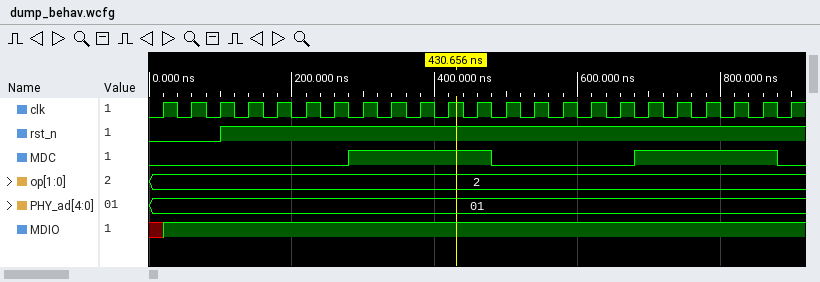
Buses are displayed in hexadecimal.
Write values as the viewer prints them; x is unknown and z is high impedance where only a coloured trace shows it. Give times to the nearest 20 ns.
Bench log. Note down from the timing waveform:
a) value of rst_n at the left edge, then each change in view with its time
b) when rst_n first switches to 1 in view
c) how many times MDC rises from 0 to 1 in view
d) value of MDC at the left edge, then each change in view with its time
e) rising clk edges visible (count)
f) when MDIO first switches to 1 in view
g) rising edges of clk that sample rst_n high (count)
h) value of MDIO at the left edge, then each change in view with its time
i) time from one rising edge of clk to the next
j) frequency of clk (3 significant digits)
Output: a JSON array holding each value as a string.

["0, 1 at 100 ns", "100 ns", "2", "0, 1 at 280 ns, 0 at 480 ns, 1 at 680 ns, 0 at 880 ns", "23", "20 ns", "20", "x, 1 at 20 ns", "40 ns", "25.0 MHz"]
